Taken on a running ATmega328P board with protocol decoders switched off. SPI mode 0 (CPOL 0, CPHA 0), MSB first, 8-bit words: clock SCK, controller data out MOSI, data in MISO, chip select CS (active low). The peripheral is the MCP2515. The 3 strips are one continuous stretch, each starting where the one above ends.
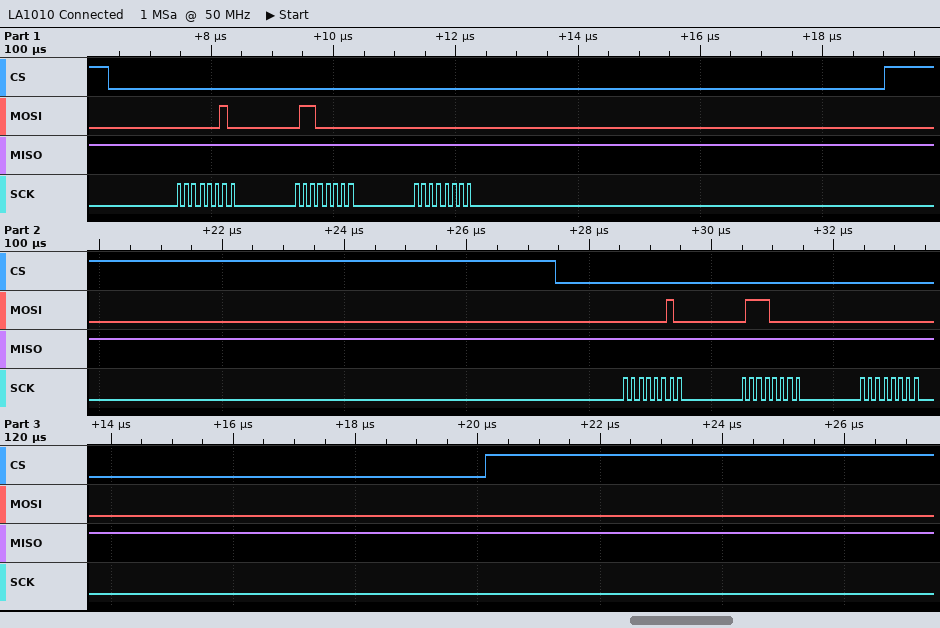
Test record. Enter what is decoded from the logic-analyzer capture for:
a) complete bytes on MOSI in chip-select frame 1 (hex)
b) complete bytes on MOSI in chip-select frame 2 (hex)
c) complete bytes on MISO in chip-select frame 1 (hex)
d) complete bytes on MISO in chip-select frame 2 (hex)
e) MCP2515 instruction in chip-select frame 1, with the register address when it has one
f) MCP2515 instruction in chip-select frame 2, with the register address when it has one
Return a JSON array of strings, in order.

["0x02 0x60 0x00", "0x02 0x70 0x00", "0xFF 0xFF 0xFF", "0xFF 0xFF 0xFF", "WRITE 0x60", "WRITE 0x70"]
